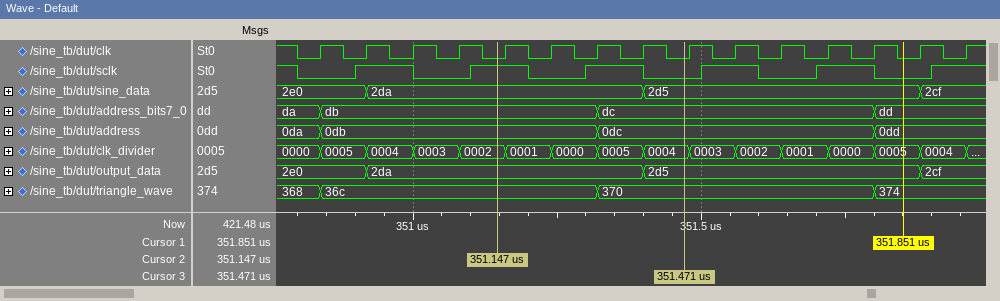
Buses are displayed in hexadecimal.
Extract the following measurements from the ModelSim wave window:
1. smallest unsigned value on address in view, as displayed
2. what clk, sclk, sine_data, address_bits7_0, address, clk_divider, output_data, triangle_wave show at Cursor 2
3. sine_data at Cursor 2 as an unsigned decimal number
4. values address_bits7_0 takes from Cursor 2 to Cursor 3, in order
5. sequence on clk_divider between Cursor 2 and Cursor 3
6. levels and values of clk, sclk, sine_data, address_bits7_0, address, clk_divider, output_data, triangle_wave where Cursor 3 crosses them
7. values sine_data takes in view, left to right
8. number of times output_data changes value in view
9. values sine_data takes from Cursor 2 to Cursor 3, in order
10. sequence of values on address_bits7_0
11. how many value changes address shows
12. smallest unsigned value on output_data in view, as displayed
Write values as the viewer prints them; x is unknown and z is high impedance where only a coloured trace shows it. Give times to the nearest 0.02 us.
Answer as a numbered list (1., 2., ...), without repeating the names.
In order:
1. 0da
2. clk=0, sclk=1, sine_data=2da, address_bits7_0=db, address=0db, clk_divider=0002, output_data=2da, triangle_wave=36c
3. 730
4. db, dc
5. 0002, 0001, 0000, 0005, 0004
6. clk=0, sclk=0, sine_data=2d5, address_bits7_0=dc, address=0dc, clk_divider=0004, output_data=2d5, triangle_wave=370
7. 2e0, 2da, 2d5, 2cf
8. 3
9. 2da, 2d5
10. da, db, dc, dd
11. 3
12. 2cf
